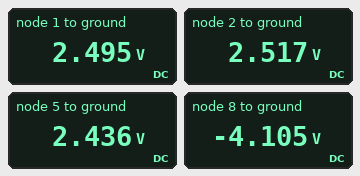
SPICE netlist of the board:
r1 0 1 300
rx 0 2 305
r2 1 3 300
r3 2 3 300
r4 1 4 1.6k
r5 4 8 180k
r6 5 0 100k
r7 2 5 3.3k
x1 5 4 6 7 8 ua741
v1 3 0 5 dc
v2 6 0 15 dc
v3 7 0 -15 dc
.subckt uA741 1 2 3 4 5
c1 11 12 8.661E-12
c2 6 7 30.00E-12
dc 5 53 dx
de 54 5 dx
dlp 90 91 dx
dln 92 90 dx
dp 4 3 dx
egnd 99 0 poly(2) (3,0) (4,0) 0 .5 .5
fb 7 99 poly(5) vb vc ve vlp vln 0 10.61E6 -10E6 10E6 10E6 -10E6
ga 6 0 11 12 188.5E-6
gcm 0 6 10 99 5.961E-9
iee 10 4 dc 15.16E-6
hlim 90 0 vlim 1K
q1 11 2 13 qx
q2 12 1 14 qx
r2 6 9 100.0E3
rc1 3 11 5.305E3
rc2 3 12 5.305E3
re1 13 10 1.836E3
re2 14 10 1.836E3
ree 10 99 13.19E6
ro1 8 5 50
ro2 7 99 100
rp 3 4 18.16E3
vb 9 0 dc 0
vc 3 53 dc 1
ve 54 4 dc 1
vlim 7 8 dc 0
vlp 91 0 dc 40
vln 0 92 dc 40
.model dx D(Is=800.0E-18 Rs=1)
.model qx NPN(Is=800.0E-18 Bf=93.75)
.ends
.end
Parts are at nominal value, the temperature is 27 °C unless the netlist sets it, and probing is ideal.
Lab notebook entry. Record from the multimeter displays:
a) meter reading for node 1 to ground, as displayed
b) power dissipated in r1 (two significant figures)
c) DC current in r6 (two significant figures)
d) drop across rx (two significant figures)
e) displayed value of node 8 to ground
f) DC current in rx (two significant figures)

2.495 V
21 mW
24 µA
2.5 V
-4.105 V
8.3 mA
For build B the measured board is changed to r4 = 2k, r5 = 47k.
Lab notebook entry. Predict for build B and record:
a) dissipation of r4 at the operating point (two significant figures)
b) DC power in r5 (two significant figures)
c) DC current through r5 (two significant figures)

1.8 µW
41 µW
30 µA
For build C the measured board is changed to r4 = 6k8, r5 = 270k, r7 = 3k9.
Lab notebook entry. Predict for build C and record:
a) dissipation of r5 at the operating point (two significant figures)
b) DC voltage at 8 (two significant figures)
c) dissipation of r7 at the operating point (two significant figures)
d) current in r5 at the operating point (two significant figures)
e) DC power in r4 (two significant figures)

33 µW
-580 mV
2.3 µW
11 µA
850 nW
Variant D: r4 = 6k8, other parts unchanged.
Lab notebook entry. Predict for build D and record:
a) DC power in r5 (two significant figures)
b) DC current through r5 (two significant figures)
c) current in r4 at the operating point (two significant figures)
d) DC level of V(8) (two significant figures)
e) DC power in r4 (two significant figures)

15 µW
9.1 µA
9.2 µA
800 mV
570 nW
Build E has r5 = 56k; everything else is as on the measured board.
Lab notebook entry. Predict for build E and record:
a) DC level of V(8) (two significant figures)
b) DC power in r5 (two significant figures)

400 mV
74 µW
